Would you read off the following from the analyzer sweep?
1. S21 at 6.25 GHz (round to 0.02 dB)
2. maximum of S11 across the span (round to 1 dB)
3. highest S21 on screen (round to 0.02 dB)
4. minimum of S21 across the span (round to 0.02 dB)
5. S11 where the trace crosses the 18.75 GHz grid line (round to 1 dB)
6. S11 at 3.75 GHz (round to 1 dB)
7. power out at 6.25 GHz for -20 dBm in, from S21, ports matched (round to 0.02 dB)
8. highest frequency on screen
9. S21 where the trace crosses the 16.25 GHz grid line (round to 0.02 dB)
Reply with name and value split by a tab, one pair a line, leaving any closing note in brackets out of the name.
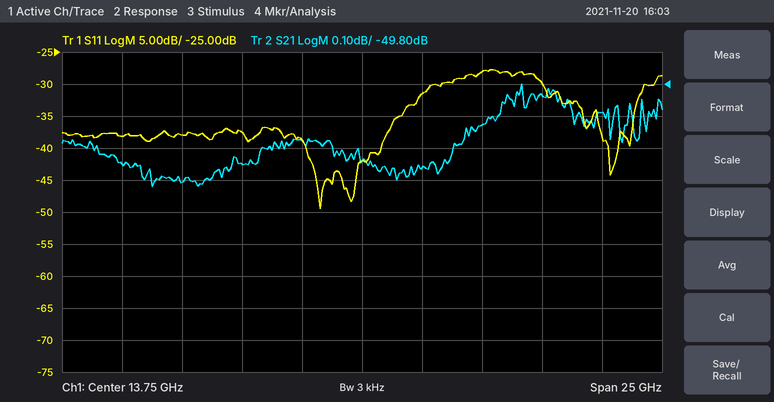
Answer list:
S21 at 6.25 GHz	-50.10 dB
maximum of S11 across the span	-28 dB
highest S21 on screen	-49.80 dB
minimum of S21 across the span	-50.12 dB
S11 where the trace crosses the 18.75 GHz grid line	-28 dB
S11 at 3.75 GHz	-38 dB
power out at 6.25 GHz for -20 dBm in, from S21, ports matched	-70.10 dBm
highest frequency on screen	26.25 GHz
S21 where the trace crosses the 16.25 GHz grid line	-50.06 dB
